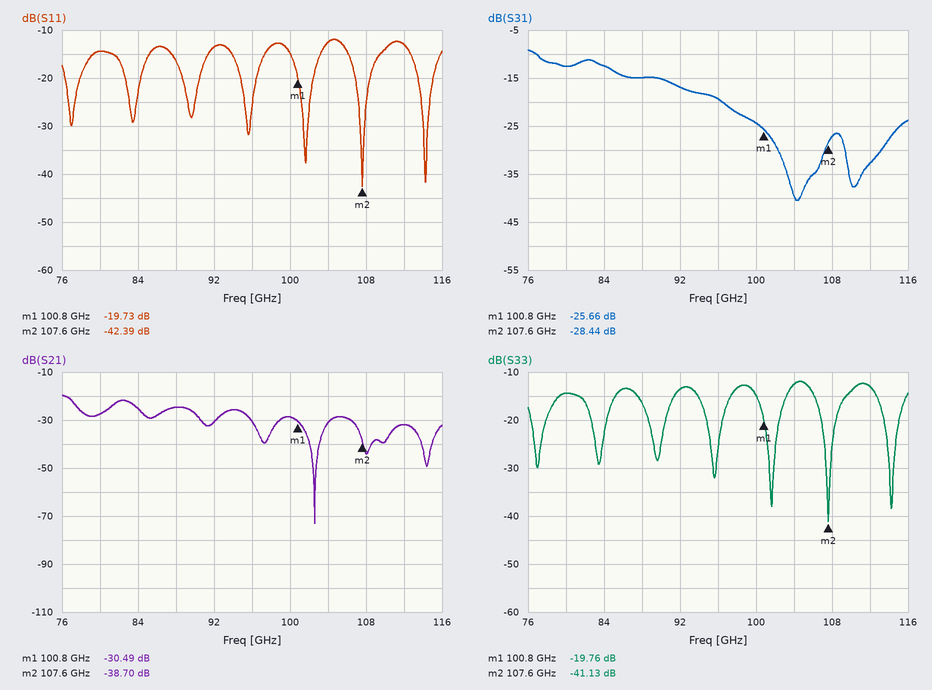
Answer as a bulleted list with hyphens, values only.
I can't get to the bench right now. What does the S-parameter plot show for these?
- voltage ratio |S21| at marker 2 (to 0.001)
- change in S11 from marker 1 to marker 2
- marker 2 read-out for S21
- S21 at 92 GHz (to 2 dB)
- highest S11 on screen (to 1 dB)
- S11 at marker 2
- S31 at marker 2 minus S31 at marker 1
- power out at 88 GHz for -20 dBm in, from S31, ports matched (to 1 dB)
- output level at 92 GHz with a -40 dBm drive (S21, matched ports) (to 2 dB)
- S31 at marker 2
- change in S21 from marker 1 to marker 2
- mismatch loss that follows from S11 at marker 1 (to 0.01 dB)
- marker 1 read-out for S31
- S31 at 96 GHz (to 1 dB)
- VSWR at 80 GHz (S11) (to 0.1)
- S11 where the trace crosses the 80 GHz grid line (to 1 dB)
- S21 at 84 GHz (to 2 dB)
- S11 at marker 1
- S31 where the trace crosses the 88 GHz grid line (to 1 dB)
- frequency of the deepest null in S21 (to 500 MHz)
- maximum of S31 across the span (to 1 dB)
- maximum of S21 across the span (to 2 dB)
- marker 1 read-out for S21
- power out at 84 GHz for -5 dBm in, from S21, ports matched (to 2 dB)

- 0.012
- -22.66 dB
- -38.70 dB
- -30 dB
- -12 dB
- -42.39 dB
- -2.78 dB
- -35 dBm
- -70 dBm
- -28.44 dB
- -8.21 dB
- 0.05 dB
- -25.66 dB
- -19 dB
- 1.5
- -14 dB
- -26 dB
- -19.73 dB
- -15 dB
- 102.5 GHz
- -9 dB
- -20 dB
- -30.49 dB
- -30 dBm
